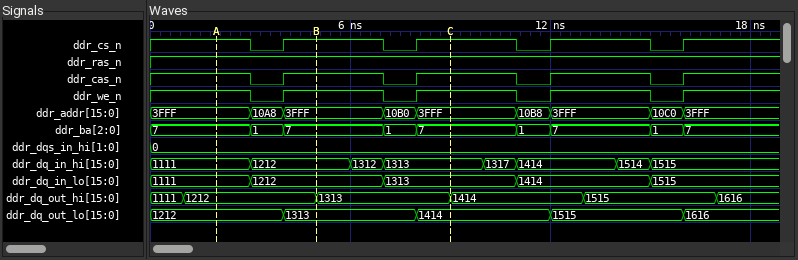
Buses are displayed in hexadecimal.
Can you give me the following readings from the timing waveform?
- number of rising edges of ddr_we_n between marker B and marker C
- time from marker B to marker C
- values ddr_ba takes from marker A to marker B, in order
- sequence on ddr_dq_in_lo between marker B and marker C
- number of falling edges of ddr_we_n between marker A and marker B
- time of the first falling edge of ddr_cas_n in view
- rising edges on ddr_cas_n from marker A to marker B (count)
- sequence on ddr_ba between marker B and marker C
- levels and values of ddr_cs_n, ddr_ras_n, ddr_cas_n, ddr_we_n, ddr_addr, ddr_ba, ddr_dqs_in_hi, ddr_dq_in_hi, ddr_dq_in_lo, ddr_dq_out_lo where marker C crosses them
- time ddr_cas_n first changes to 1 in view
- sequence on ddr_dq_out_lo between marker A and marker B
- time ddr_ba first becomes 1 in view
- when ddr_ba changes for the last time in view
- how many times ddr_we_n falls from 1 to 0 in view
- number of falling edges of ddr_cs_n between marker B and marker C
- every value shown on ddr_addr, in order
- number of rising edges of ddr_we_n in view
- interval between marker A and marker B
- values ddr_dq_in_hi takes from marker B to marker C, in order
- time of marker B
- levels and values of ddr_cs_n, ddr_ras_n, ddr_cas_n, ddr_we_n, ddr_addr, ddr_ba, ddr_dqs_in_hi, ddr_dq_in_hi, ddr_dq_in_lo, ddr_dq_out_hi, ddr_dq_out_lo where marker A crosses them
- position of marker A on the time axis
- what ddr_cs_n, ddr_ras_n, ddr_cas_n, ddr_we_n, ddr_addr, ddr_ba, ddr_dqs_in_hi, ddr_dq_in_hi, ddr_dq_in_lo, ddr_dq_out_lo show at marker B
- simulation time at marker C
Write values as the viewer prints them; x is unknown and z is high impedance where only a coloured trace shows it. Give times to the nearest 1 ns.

1
4 ns
7, 1, 7
1212, 1313
1
3 ns
1
7, 1, 7
ddr_cs_n=1, ddr_ras_n=1, ddr_cas_n=1, ddr_we_n=1, ddr_addr=3FFF, ddr_ba=7, ddr_dqs_in_hi=0, ddr_dq_in_hi=1313, ddr_dq_in_lo=1313, ddr_dq_out_lo=1414
4 ns
1212, 1313
3 ns
16 ns
4
1
3FFF, 10A8, 3FFF, 10B0, 3FFF, 10B8, 3FFF, 10C0, 3FFF
4
3 ns
1212, 1312, 1313
5 ns
ddr_cs_n=1, ddr_ras_n=1, ddr_cas_n=1, ddr_we_n=1, ddr_addr=3FFF, ddr_ba=7, ddr_dqs_in_hi=0, ddr_dq_in_hi=1111, ddr_dq_in_lo=1111, ddr_dq_out_hi=1212, ddr_dq_out_lo=1212
2 ns
ddr_cs_n=1, ddr_ras_n=1, ddr_cas_n=1, ddr_we_n=1, ddr_addr=3FFF, ddr_ba=7, ddr_dqs_in_hi=0, ddr_dq_in_hi=1212, ddr_dq_in_lo=1212, ddr_dq_out_lo=1313
9 ns
